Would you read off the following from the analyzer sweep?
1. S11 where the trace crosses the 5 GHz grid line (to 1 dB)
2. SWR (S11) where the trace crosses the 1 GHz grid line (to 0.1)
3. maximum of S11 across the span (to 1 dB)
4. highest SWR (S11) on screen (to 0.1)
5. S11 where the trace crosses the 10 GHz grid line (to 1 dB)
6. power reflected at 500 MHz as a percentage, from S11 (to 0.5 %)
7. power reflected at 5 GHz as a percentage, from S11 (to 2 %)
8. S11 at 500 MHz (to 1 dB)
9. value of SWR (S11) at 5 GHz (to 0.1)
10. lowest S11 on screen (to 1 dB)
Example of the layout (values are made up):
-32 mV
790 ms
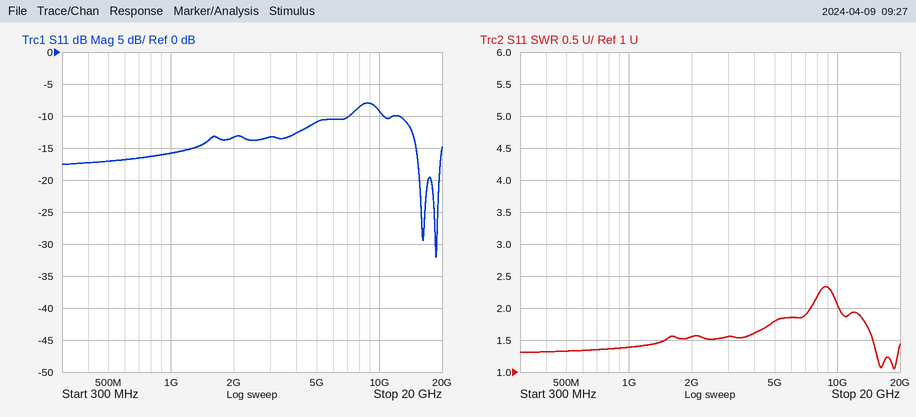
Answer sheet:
-11 dB
1.4
-8 dB
2.3
-9 dB
2.0 %
8 %
-17 dB
1.8
-32 dB
